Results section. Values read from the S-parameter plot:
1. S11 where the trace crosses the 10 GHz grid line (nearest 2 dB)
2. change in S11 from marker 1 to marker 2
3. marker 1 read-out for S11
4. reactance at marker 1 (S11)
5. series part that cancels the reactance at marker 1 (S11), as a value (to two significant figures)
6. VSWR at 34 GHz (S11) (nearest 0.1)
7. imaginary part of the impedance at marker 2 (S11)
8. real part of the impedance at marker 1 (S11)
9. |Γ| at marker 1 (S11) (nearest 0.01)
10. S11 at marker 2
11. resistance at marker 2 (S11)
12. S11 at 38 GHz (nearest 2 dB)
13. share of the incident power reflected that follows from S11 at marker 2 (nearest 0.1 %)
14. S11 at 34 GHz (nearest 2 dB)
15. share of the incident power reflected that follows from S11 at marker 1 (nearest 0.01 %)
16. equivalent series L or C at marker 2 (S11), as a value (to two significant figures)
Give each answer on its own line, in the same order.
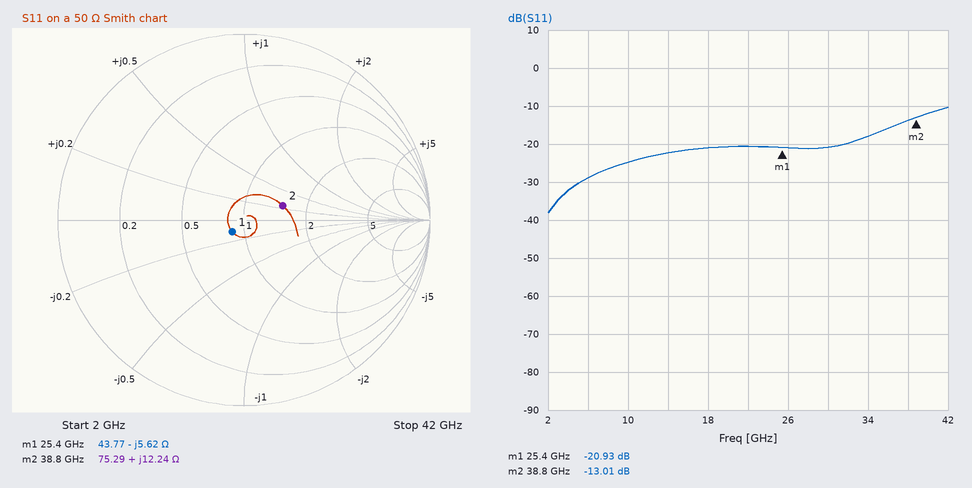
-24 dB
7.92 dB
-20.93 dB
-5.62 Ω
35 pH
1.3
+12.24 Ω
43.77 Ω
0.09
-13.01 dB
75.29 Ω
-14 dB
5.0 %
-18 dB
0.81 %
50 pH
